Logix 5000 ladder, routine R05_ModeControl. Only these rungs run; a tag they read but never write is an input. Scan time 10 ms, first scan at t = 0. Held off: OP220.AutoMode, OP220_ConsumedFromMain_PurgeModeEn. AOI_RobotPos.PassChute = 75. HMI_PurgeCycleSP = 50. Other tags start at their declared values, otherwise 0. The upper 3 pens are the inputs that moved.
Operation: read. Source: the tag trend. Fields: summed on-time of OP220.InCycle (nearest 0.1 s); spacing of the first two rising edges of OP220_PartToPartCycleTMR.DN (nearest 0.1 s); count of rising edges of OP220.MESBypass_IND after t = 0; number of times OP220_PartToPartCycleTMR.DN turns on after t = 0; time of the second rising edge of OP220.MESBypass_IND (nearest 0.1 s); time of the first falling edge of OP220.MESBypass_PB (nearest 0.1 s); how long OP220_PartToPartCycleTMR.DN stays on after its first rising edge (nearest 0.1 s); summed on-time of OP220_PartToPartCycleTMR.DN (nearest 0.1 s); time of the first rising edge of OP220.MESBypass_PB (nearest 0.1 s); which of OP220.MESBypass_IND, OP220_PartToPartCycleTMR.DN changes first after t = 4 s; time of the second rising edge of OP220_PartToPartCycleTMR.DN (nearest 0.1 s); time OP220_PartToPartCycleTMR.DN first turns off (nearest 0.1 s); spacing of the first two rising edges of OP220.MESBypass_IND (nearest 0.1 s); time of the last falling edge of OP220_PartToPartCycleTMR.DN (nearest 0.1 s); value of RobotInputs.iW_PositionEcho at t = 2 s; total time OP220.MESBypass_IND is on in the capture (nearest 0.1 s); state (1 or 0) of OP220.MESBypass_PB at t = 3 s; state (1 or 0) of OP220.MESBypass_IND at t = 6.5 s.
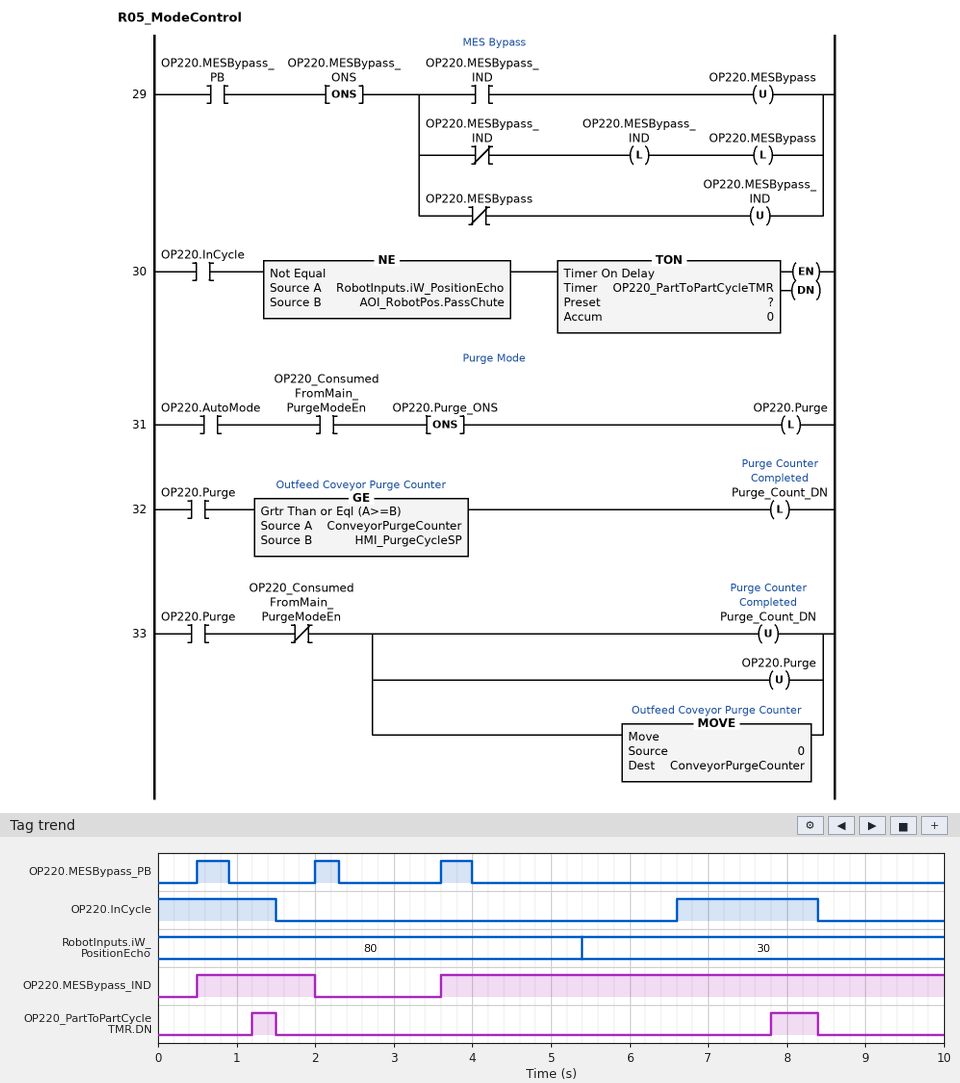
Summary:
3.3 s
6.6 s
2
2
3.6 s
0.9 s
0.3 s
0.9 s
0.5 s
OP220_PartToPartCycleTMR.DN
7.8 s
1.5 s
3.1 s
8.4 s
80
7.9 s
0
1
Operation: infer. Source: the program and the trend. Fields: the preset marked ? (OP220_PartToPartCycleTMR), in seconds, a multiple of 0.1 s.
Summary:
1.2 s
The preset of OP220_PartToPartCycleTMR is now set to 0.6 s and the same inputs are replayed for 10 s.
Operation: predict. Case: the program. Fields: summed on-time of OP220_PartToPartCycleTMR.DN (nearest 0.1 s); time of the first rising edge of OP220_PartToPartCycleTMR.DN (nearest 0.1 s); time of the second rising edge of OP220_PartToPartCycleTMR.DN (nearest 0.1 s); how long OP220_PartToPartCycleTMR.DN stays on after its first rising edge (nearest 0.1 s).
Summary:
2.1 s
0.6 s
7.2 s
0.9 s
